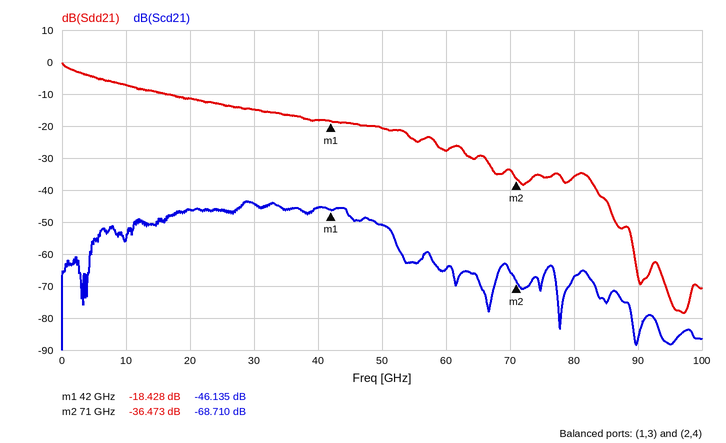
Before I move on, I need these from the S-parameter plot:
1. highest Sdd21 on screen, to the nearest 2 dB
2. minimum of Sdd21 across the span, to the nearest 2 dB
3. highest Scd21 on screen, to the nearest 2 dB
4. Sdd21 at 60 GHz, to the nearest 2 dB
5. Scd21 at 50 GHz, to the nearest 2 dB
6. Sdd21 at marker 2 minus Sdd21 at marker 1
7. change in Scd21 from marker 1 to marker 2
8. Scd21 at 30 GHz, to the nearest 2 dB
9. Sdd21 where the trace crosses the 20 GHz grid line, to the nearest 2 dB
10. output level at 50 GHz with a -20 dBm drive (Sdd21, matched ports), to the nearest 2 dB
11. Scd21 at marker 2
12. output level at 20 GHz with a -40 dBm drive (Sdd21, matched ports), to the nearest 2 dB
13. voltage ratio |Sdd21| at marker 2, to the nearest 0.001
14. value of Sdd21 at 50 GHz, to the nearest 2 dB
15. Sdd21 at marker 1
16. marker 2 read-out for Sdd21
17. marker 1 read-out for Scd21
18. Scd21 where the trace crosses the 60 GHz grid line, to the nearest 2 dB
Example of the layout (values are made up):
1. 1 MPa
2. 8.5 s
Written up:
1. 0 dB
2. -78 dB
3. -44 dB
4. -28 dB
5. -50 dB
6. -18.045 dB
7. -22.575 dB
8. -44 dB
9. -12 dB
10. -40 dBm
11. -68.710 dB
12. -52 dBm
13. 0.015
14. -20 dB
15. -18.428 dB
16. -36.473 dB
17. -46.135 dB
18. -64 dB
